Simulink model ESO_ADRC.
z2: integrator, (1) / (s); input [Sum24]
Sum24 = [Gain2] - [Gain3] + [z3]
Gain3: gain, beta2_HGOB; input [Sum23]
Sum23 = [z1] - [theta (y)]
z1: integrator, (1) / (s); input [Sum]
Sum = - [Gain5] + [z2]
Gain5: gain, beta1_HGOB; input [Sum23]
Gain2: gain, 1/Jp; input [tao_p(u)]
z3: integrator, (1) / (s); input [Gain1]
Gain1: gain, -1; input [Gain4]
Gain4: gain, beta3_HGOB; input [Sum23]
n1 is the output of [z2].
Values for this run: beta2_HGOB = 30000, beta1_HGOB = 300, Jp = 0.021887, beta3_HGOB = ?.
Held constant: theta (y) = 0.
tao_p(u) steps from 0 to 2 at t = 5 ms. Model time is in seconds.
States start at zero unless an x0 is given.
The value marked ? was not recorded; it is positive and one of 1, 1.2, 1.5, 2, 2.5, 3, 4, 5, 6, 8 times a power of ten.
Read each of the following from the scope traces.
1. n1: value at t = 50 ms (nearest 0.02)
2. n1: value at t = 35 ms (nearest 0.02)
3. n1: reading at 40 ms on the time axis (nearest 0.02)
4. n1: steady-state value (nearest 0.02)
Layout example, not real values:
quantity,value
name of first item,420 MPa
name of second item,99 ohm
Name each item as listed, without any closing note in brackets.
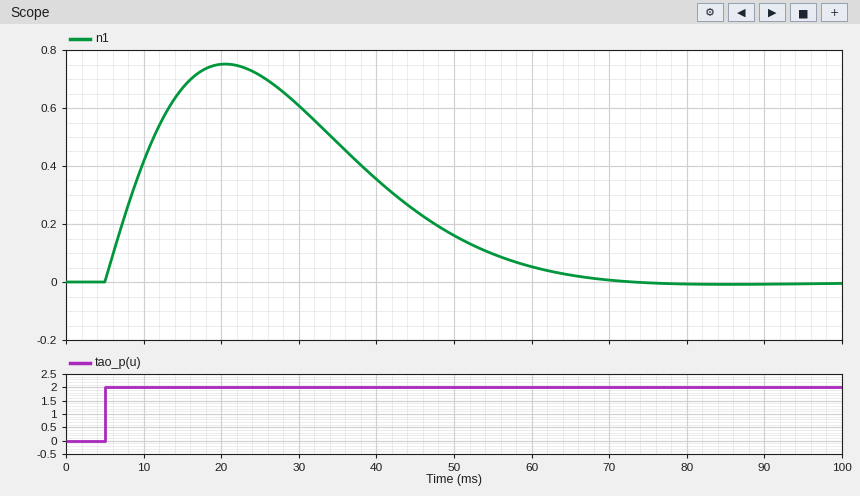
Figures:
quantity,value
n1: value at t = 50 ms,0.16
n1: value at t = 35 ms,0.48
n1: reading at 40 ms on the time axis,0.36
n1: steady-state value,0.00
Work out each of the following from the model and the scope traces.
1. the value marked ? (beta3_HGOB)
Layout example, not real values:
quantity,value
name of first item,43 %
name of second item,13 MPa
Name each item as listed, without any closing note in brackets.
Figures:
quantity,value
the value marked ?,1.2e+06
